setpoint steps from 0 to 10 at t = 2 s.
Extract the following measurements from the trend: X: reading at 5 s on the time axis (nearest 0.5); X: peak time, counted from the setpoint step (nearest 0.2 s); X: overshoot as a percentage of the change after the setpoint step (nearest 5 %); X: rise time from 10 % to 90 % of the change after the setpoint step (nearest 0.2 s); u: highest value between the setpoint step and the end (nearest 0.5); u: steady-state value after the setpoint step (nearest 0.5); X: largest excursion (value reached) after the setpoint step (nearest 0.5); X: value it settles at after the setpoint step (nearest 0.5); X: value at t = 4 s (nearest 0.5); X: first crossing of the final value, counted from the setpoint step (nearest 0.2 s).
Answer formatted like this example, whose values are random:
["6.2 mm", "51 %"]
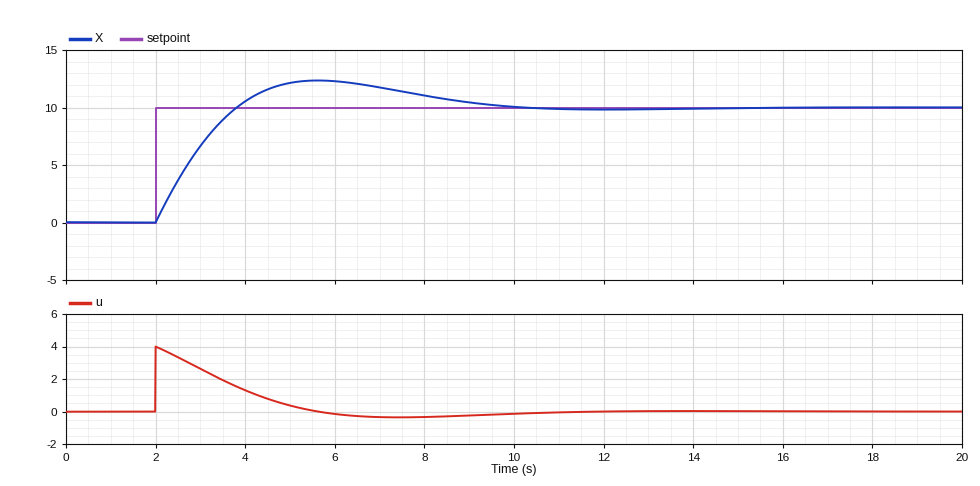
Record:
["12.0", "3.6 s", "25 %", "1.4 s", "4.0", "0.0", "12.5", "10.0", "10.5", "1.8 s"]
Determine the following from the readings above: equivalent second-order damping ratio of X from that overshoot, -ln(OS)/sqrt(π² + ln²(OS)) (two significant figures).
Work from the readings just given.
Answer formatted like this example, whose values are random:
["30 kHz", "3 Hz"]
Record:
["0.40"]
